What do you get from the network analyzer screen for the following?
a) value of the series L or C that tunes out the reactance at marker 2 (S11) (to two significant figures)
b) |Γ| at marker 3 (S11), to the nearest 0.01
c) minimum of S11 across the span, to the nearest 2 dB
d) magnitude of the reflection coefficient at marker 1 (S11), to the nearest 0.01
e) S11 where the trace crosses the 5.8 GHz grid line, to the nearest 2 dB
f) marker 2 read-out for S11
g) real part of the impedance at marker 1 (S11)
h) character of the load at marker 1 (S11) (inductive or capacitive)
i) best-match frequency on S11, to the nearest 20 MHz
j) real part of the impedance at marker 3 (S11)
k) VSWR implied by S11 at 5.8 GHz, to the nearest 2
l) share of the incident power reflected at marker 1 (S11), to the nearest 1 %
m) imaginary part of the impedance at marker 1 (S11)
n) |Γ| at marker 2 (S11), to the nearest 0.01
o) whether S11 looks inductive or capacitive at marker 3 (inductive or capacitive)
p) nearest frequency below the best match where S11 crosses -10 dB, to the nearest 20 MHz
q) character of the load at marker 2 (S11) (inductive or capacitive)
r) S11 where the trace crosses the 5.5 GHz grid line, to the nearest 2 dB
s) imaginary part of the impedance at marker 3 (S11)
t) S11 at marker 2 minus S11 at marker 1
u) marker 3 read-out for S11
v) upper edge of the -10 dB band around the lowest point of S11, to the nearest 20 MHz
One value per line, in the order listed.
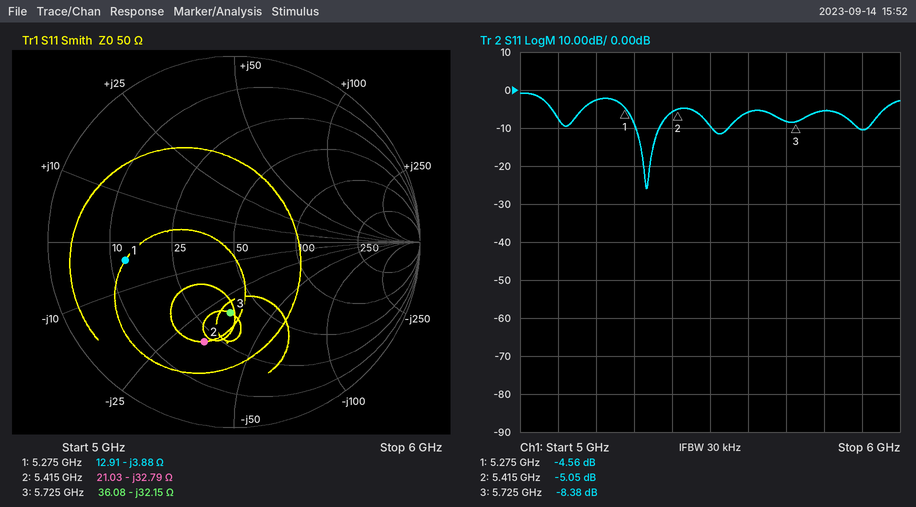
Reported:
960 pH
0.38
-26 dB
0.59
-6 dB
-5.05 dB
12.91 Ω
capacitive
5.34 GHz
36.08 Ω
4
35 %
-3.88 Ω
0.56
capacitive
5.30 GHz
capacitive
-10 dB
-32.15 Ω
-0.49 dB
-8.38 dB
5.36 GHz
